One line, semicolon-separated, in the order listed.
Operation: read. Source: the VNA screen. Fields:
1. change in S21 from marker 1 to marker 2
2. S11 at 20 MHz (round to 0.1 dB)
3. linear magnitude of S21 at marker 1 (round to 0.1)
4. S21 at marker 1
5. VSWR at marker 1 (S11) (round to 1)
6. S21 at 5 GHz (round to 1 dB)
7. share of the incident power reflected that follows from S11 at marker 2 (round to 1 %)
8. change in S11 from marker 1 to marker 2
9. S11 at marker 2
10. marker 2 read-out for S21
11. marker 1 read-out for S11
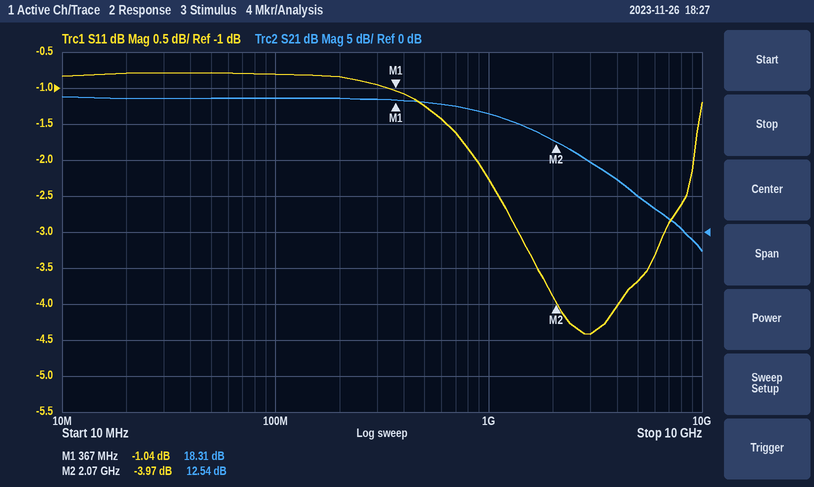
-5.77 dB; -0.8 dB; 8.2; 18.31 dB; 17; 5 dB; 40 %; -2.93 dB; -3.97 dB; 12.54 dB; -1.04 dB
